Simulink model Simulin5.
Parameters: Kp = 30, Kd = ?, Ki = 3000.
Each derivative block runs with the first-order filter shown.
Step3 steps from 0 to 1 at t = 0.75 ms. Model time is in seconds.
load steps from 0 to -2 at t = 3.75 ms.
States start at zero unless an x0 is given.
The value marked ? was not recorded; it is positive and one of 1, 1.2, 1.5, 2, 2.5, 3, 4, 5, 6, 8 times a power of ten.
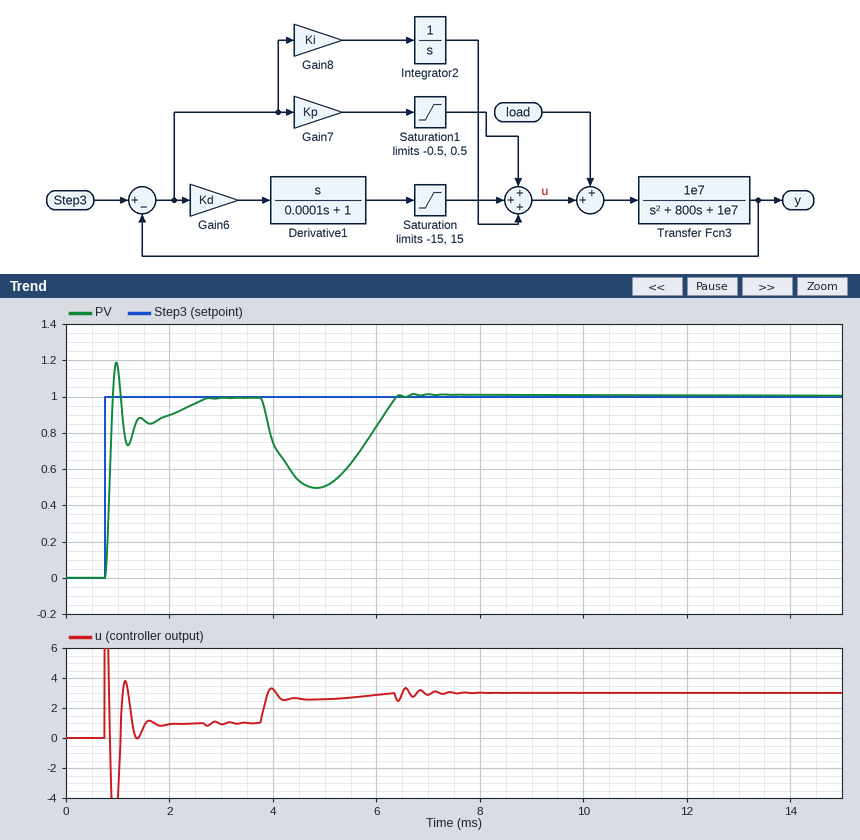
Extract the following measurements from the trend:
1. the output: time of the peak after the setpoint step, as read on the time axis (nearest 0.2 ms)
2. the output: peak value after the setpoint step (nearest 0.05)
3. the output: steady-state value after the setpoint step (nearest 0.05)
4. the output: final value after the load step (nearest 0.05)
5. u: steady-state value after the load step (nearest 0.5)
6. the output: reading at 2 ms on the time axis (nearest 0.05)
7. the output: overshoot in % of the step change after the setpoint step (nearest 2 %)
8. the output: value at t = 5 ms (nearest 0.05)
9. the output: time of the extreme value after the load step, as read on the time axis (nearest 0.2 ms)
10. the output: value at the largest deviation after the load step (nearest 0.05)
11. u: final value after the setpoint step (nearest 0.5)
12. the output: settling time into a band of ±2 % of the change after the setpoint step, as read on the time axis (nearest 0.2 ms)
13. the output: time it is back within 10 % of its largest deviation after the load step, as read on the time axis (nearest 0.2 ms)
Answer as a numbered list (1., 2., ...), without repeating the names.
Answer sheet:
1. 1.0 ms
2. 1.20
3. 1.00
4. 1.00
5. 3.0
6. 0.90
7. 18 %
8. 0.50
9. 4.8 ms
10. 0.50
11. 1.0
12. 2.6 ms
13. 6.2 ms
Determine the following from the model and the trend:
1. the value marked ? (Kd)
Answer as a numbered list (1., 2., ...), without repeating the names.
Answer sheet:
1. 0.002
